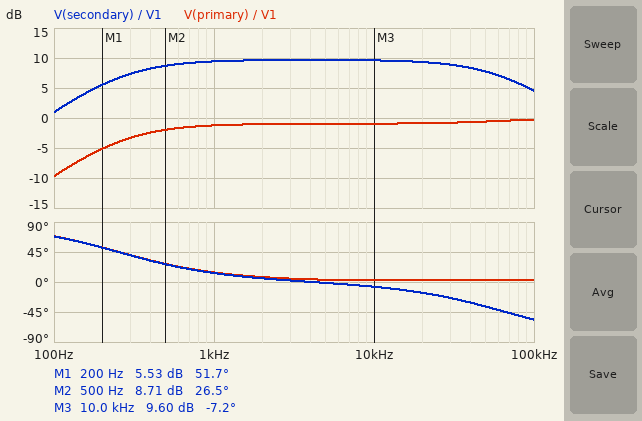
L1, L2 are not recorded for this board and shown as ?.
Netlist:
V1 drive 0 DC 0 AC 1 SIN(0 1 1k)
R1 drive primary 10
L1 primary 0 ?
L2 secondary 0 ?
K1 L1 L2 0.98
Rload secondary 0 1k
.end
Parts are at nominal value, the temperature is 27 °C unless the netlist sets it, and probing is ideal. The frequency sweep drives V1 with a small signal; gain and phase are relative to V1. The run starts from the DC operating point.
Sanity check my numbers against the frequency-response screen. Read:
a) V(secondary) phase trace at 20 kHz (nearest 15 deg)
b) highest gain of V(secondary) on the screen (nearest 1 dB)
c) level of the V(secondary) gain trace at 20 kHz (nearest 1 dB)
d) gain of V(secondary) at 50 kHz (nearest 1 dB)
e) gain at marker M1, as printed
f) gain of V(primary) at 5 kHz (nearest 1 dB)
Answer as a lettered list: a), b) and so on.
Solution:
a) -15 deg
b) 10 dB
c) 9 dB
d) 8 dB
e) 5.53 dB
f) -1 dB
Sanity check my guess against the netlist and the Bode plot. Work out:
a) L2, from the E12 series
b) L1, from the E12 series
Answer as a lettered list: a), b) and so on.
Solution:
a) 68 mH
b) 5.6 mH
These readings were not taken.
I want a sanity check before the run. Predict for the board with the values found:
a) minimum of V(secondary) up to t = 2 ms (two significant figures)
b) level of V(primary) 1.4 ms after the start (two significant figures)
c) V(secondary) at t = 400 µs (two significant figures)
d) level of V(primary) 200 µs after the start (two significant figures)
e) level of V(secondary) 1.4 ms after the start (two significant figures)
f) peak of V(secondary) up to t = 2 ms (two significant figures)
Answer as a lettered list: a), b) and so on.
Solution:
a) -3.2 V
b) 300 mV
c) 750 mV
d) 710 mV
e) 1.1 V
f) 2.9 V
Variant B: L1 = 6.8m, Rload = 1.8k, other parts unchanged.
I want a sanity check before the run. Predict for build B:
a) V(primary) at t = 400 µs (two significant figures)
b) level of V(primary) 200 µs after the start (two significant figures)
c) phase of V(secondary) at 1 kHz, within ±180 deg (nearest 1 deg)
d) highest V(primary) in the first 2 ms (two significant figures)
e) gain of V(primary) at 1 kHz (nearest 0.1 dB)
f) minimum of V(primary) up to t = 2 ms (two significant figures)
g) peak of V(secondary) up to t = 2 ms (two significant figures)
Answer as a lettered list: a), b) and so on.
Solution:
a) 250 mV
b) 770 mV
c) 12 deg
d) 890 mV
e) -0.7 dB
f) -1.0 V
g) 2.8 V
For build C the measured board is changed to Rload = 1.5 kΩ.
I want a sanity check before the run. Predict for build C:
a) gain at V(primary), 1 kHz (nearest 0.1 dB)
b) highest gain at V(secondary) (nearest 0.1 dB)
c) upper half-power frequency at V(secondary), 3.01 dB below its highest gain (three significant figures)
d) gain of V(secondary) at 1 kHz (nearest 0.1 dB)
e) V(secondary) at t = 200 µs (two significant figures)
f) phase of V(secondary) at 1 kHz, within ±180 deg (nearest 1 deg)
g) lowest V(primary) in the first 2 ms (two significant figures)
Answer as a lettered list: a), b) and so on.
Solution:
a) -0.9 dB
b) 10.0 dB
c) 96.1 kHz
d) 9.7 dB
e) 2.5 V
f) 14 deg
g) -970 mV
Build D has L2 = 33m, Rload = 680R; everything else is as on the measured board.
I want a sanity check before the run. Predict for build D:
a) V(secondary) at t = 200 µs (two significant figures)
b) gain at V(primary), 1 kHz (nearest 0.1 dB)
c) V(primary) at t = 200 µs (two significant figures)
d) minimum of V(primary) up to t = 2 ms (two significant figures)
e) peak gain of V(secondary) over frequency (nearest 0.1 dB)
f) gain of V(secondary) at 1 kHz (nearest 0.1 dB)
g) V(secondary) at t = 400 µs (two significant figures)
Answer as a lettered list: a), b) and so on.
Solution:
a) 1.7 V
b) -1.0 dB
c) 730 mV
d) -960 mV
e) 6.8 dB
f) 6.5 dB
g) 510 mV
